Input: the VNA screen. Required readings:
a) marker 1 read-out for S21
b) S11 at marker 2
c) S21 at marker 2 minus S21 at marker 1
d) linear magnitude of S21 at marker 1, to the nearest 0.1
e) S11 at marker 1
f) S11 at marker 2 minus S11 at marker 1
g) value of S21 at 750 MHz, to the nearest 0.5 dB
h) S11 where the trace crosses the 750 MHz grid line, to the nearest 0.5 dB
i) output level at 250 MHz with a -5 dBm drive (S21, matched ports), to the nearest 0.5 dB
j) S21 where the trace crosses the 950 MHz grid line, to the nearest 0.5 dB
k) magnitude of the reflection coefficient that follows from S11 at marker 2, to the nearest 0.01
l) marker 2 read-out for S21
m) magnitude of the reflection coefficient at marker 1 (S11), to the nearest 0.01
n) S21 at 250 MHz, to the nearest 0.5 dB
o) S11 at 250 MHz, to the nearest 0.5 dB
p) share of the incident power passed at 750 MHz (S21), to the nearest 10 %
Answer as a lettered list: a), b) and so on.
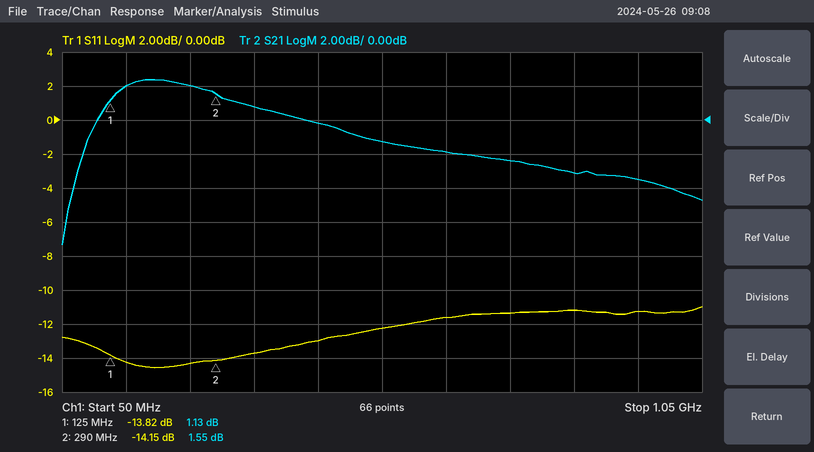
a) 1.13 dB
b) -14.15 dB
c) 0.42 dB
d) 1.1
e) -13.82 dB
f) -0.33 dB
g) -2.5 dB
h) -11.5 dB
i) -3.0 dBm
j) -3.5 dB
k) 0.20
l) 1.55 dB
m) 0.20
n) 2.0 dB
o) -14.5 dB
p) 60 %
